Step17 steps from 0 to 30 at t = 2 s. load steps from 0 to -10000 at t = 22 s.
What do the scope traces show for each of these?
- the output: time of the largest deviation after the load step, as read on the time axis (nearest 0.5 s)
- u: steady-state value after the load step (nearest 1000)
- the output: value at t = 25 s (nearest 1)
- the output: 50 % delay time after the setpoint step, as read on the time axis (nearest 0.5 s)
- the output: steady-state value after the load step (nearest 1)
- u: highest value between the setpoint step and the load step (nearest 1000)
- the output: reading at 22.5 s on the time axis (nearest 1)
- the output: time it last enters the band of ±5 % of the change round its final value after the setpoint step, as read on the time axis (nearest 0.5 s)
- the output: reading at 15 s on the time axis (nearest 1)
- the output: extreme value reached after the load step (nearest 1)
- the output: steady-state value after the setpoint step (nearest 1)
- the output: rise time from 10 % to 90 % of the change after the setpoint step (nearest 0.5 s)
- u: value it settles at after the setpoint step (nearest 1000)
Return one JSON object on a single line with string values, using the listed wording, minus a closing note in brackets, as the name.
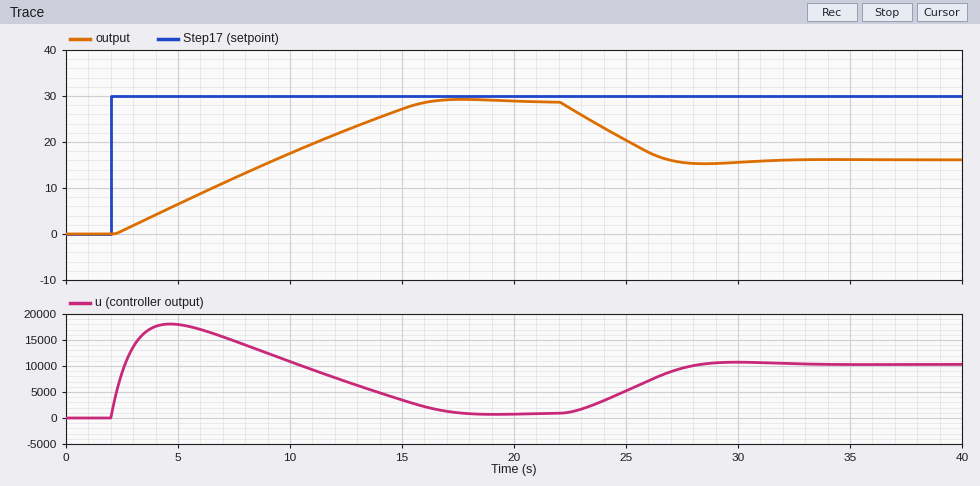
{"the output: time of the largest deviation after the load step, as read on the time axis": "28.5 s", "u: steady-state value after the load step": "10000", "the output: value at t = 25 s": "20", "the output: 50 % delay time after the setpoint step, as read on the time axis": "8.5 s", "the output: steady-state value after the load step": "16", "u: highest value between the setpoint step and the load step": "18000", "the output: reading at 22.5 s on the time axis": "27", "the output: time it last enters the band of ±5 % of the change round its final value after the setpoint step, as read on the time axis": "15.0 s", "the output: reading at 15 s on the time axis": "27", "the output: extreme value reached after the load step": "15", "the output: steady-state value after the setpoint step": "29", "the output: rise time from 10 % to 90 % of the change after the setpoint step": "11.0 s", "u: value it settles at after the setpoint step": "1000"}
